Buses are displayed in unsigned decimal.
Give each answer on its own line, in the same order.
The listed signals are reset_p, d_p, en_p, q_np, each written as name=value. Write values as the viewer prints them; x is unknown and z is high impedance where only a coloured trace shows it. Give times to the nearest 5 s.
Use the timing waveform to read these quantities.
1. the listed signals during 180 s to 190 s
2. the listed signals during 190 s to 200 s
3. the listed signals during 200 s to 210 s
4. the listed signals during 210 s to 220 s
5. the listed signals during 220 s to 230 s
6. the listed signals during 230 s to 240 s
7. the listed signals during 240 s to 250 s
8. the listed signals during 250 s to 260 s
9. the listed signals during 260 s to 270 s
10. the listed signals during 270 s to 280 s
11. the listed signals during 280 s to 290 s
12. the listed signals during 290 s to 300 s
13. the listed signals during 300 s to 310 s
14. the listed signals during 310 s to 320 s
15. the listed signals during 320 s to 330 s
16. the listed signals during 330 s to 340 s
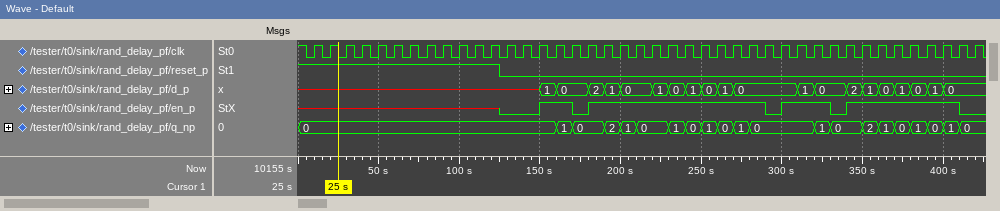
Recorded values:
reset_p=0, d_p=2, en_p=1, q_np=0
reset_p=0, d_p=1, en_p=1, q_np=2
reset_p=0, d_p=0, en_p=1, q_np=1
reset_p=0, d_p=0, en_p=1, q_np=0
reset_p=0, d_p=1, en_p=1, q_np=0
reset_p=0, d_p=0, en_p=1, q_np=1
reset_p=0, d_p=1, en_p=1, q_np=0
reset_p=0, d_p=0, en_p=1, q_np=1
reset_p=0, d_p=1, en_p=1, q_np=0
reset_p=0, d_p=0, en_p=1, q_np=1
reset_p=0, d_p=0, en_p=1, q_np=0
reset_p=0, d_p=0, en_p=0, q_np=0
reset_p=0, d_p=0, en_p=1, q_np=0
reset_p=0, d_p=1, en_p=1, q_np=0
reset_p=0, d_p=0, en_p=1, q_np=1
reset_p=0, d_p=0, en_p=0, q_np=0
